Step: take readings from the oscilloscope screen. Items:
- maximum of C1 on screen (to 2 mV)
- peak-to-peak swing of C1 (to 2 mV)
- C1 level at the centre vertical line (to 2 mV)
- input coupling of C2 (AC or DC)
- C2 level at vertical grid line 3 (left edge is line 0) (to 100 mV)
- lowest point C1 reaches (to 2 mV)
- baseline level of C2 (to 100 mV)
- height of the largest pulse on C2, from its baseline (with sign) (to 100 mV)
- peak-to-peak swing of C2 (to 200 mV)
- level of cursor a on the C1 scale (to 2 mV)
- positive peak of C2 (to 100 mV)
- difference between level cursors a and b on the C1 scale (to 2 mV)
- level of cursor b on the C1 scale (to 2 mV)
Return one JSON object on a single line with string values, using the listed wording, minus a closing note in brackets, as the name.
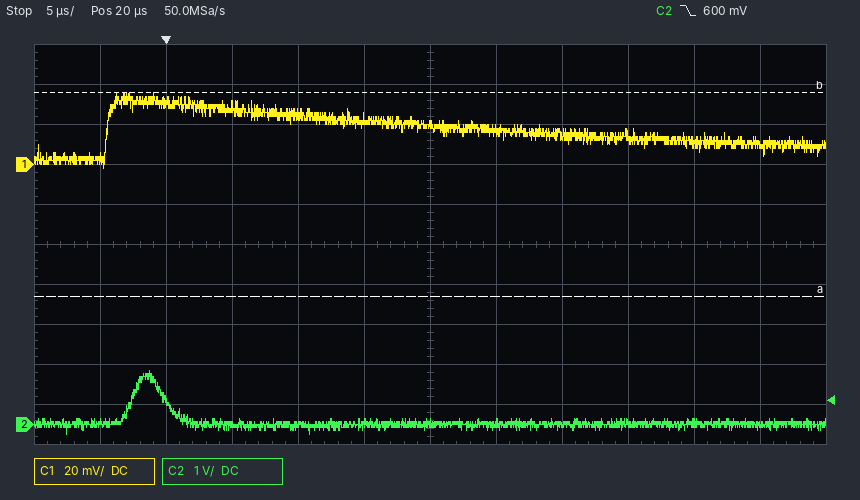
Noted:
{"maximum of C1 on screen": "36 mV", "peak-to-peak swing of C1": "38 mV", "C1 level at the centre vertical line": "20 mV", "input coupling of C2": "DC", "C2 level at vertical grid line 3 (left edge is line 0)": "0.0 V", "lowest point C1 reaches": "-2 mV", "baseline level of C2": "0.0 V", "height of the largest pulse on C2, from its baseline (with sign)": "+1.4 V", "peak-to-peak swing of C2": "1.6 V", "level of cursor a on the C1 scale": "-66 mV", "positive peak of C2": "1.4 V", "difference between level cursors a and b on the C1 scale": "102 mV", "level of cursor b on the C1 scale": "36 mV"}
